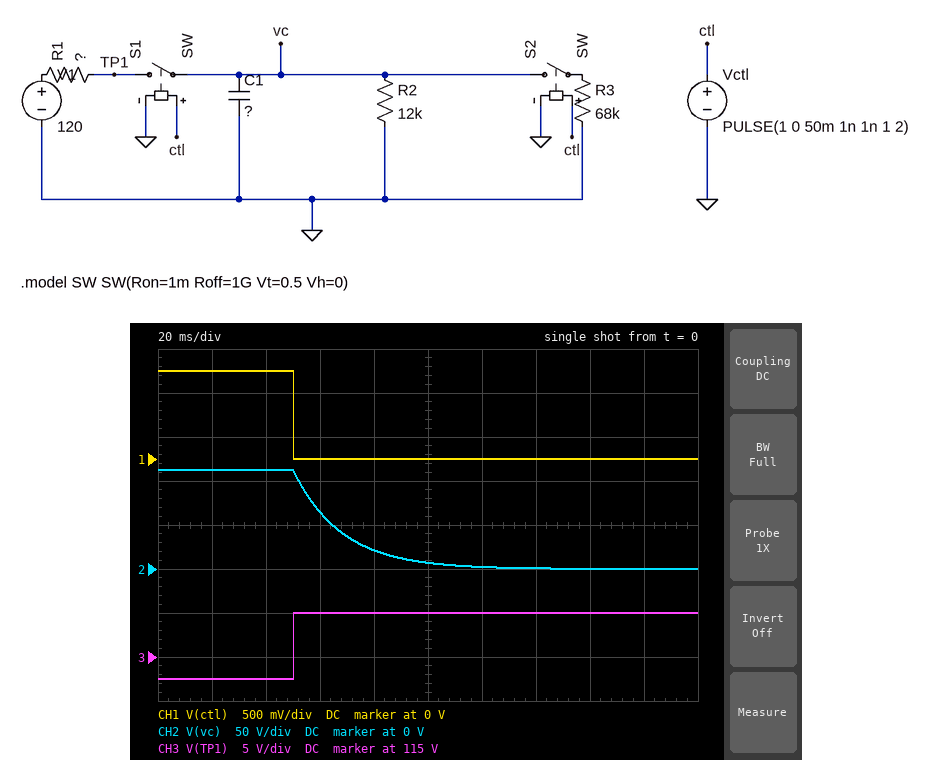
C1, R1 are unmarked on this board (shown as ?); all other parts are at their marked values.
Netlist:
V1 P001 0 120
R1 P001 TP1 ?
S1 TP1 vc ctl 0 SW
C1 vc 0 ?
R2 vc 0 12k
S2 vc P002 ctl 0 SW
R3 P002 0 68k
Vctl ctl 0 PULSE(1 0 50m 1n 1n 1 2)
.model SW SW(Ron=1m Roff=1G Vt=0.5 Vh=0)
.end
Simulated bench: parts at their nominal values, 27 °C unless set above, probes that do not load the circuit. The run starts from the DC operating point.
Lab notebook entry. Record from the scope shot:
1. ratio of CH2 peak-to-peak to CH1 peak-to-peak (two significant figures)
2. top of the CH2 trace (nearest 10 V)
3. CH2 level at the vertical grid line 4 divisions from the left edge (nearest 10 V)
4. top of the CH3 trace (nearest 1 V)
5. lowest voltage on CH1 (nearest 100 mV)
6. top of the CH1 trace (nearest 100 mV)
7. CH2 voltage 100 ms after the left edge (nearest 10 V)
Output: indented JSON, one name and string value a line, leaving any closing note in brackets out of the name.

{
  "ratio of CH2 peak-to-peak to CH1 peak-to-peak": "110",
  "top of the CH2 trace": "110 V",
  "CH2 level at the vertical grid line 4 divisions from the left edge": "20 V",
  "top of the CH3 trace": "120 V",
  "lowest voltage on CH1": "0 V",
  "top of the CH1 trace": "1.0 V",
  "CH2 voltage 100 ms after the left edge": "10 V"
}
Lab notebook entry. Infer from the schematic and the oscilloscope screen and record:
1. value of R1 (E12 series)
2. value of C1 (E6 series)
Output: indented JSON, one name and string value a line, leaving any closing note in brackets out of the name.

{
  "value of R1": "680 Ω",
  "value of C1": "1.5 µF"
}
